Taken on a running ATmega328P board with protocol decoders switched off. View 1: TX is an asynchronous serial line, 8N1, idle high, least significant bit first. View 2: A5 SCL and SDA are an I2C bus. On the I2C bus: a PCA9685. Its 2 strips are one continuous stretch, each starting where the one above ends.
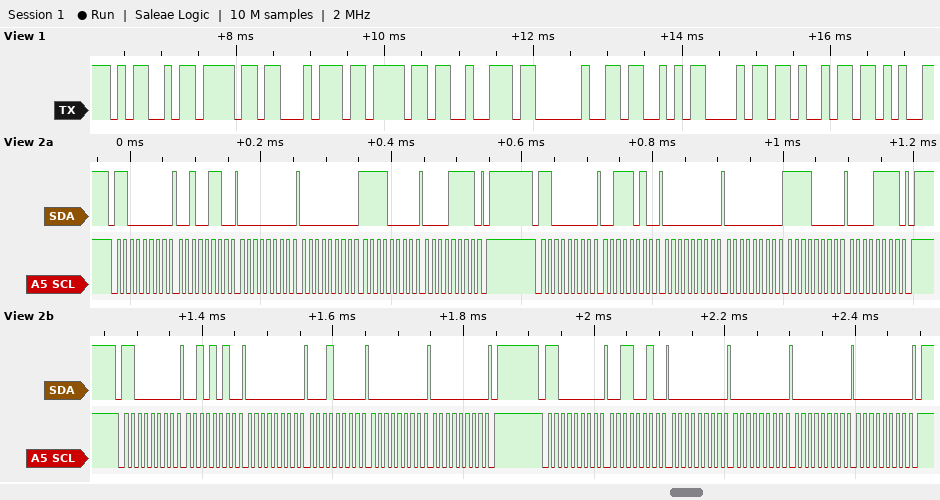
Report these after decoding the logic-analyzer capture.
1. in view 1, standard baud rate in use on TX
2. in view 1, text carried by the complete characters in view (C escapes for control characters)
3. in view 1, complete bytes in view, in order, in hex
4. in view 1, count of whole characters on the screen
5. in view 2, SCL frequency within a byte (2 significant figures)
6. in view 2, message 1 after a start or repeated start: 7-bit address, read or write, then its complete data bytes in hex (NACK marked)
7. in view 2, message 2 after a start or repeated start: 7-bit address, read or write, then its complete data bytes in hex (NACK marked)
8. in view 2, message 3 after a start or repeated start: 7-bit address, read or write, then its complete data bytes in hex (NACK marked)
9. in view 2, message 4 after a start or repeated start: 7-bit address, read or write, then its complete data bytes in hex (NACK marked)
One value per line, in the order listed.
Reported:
9600 baud
"Motor Shi"
4D 6F 74 6F 72 20 53 68 69
9
100 kHz
0x60 write: 26 00 00 F0 0F
0x60 write: 3A 00 00 F0 0F
0x60 write: 2A 00 10 00 00
0x60 write: 32 00 00 00 00
